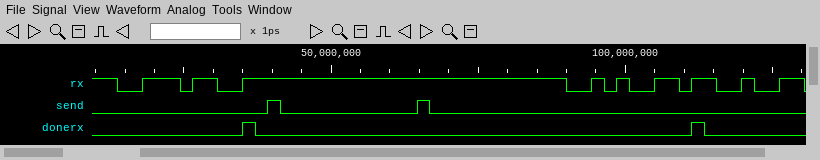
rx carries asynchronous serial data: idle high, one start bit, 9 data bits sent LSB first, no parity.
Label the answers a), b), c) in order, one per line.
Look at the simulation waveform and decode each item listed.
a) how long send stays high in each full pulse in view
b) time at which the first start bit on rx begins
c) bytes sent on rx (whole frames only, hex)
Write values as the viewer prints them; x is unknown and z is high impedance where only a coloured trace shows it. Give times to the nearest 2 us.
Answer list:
a) 2 us, 2 us
b) 14 us
c) 6E, CA
